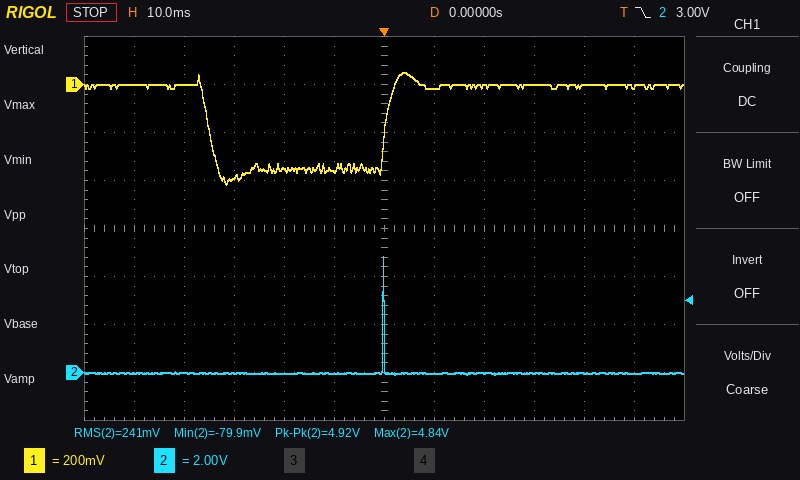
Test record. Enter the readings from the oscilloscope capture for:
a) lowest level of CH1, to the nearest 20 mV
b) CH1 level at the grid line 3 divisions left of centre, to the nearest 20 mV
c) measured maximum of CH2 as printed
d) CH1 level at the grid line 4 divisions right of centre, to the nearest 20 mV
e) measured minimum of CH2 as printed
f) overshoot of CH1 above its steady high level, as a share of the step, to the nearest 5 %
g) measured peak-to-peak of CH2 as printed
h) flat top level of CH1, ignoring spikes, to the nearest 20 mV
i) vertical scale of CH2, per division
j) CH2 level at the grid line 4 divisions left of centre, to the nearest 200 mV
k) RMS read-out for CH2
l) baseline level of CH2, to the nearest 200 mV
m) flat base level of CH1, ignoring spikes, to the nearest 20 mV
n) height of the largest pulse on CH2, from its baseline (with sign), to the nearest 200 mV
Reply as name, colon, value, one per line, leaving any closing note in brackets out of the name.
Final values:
lowest level of CH1, to the nearest 20 mV: -420 mV
CH1 level at the grid line 3 divisions left of centre, to the nearest 20 mV: -380 mV
measured maximum of CH2 as printed: 4.84 V
CH1 level at the grid line 4 divisions right of centre, to the nearest 20 mV: 0 mV
measured minimum of CH2 as printed: -79.9 mV
overshoot of CH1 above its steady high level, as a share of the step, to the nearest 5 %: 15 %
measured peak-to-peak of CH2 as printed: 4.92 V
flat top level of CH1, ignoring spikes, to the nearest 20 mV: 0 mV
vertical scale of CH2, per division: 2 V
CH2 level at the grid line 4 divisions left of centre, to the nearest 200 mV: 0.0 V
RMS read-out for CH2: 241 mV
baseline level of CH2, to the nearest 200 mV: 0.0 V
flat base level of CH1, ignoring spikes, to the nearest 20 mV: -360 mV
height of the largest pulse on CH2, from its baseline (with sign), to the nearest 200 mV: +4.8 V
